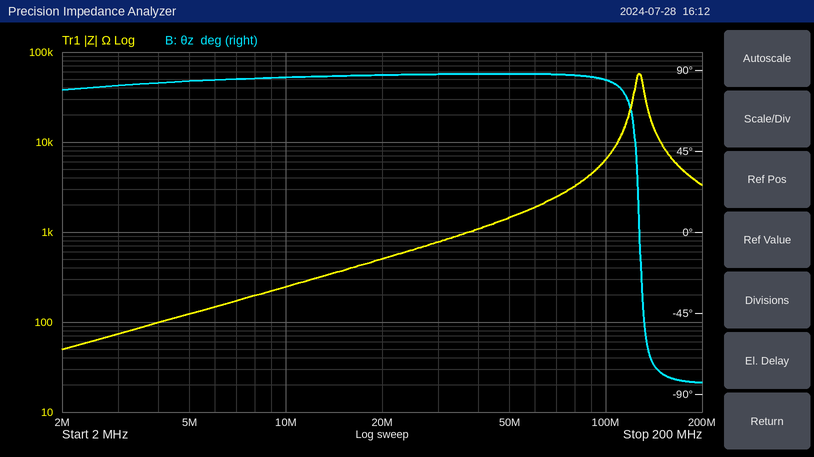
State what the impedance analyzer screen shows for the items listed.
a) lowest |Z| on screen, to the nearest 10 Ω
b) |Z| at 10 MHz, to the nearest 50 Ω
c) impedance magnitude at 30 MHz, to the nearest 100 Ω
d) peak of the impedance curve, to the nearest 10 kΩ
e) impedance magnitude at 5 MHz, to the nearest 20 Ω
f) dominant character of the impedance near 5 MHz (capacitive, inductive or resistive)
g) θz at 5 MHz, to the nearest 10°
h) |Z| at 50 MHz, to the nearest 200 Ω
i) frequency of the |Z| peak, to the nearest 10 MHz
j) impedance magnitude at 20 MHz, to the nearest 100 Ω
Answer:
50 Ω
250 Ω
800 Ω
60 kΩ
120 Ω
inductive
80°
1.4 kΩ
130 MHz
500 Ω
